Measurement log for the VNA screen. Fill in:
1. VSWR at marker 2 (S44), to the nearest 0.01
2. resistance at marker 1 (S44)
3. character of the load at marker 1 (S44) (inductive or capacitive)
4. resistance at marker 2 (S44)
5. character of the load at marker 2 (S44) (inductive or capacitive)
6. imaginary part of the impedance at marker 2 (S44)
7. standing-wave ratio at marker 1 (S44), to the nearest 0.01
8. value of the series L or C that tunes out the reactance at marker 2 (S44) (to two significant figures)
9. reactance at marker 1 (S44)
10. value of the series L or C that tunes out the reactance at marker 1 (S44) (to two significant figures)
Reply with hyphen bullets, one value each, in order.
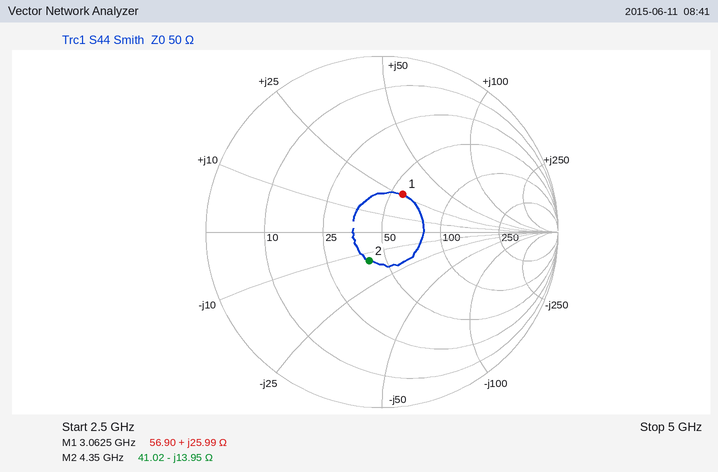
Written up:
- 1.44
- 56.90 Ω
- inductive
- 41.02 Ω
- capacitive
- -13.95 Ω
- 1.65
- 510 pH
- +25.99 Ω
- 2.0 pF
